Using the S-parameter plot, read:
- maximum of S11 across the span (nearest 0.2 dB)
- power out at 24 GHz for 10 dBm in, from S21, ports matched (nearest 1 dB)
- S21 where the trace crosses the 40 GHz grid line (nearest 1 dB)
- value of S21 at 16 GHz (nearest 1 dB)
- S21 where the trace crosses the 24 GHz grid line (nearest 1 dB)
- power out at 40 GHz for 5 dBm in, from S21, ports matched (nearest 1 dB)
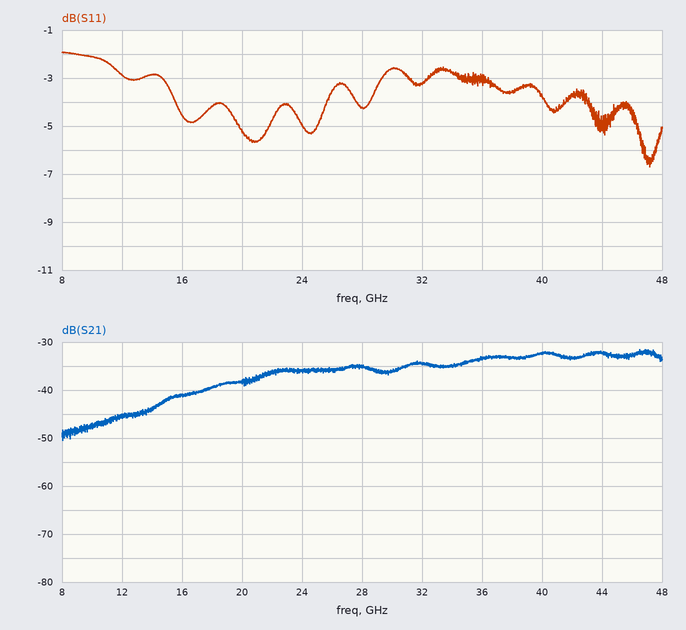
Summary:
-2.0 dB
-26 dBm
-32 dB
-41 dB
-36 dB
-27 dBm
